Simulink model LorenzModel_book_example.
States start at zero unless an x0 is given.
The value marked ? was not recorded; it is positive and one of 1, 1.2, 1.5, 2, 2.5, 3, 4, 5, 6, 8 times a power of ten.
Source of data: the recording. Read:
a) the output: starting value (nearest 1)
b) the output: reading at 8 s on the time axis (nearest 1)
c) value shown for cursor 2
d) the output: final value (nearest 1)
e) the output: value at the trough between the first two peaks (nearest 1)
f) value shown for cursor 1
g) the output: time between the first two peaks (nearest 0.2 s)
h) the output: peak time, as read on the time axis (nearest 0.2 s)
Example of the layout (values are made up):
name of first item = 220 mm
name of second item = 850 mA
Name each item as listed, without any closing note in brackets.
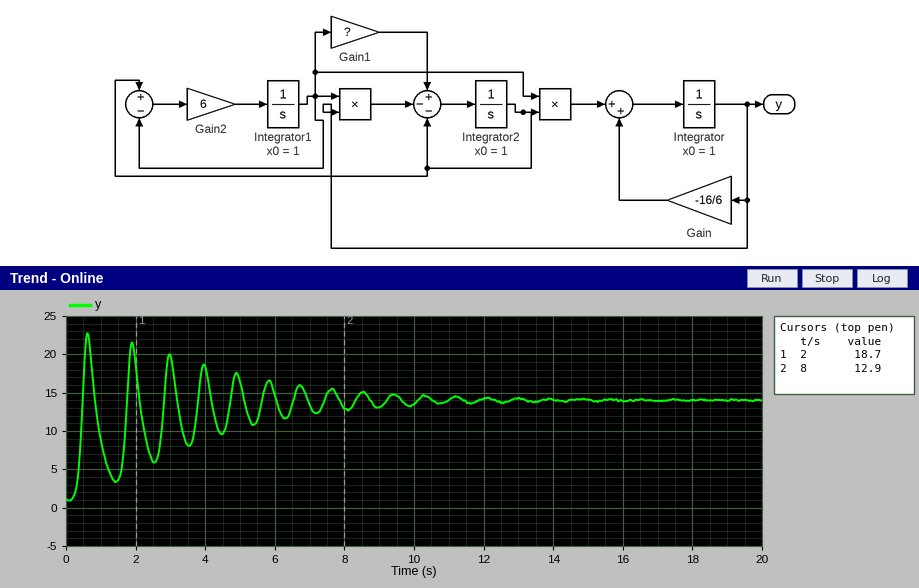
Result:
the output: starting value = 1
the output: reading at 8 s on the time axis = 13
value shown for cursor 2 = 12.9
the output: final value = 14
the output: value at the trough between the first two peaks = 3
value shown for cursor 1 = 18.7
the output: time between the first two peaks = 1.2 s
the output: peak time, as read on the time axis = 0.6 s
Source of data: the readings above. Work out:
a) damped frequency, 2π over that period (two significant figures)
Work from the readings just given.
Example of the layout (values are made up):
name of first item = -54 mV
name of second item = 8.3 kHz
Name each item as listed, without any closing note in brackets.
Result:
damped frequency, 2π over that period = 5.2 rad/s
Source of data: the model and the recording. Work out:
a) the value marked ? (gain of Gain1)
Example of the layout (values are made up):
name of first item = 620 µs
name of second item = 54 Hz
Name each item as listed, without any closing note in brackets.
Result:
the value marked ? = 15
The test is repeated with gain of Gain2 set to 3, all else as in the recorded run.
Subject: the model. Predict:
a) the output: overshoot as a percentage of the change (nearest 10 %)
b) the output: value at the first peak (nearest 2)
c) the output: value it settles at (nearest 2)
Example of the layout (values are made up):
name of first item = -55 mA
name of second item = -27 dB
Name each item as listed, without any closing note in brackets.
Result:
the output: overshoot as a percentage of the change = 60 %
the output: value at the first peak = 22
the output: value it settles at = 14
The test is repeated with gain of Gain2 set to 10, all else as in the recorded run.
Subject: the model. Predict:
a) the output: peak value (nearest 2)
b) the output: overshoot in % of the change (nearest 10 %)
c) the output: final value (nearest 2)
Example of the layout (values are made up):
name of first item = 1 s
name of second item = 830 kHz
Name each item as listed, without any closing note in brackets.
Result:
the output: peak value = 24
the output: overshoot in % of the change = 70 %
the output: final value = 14
